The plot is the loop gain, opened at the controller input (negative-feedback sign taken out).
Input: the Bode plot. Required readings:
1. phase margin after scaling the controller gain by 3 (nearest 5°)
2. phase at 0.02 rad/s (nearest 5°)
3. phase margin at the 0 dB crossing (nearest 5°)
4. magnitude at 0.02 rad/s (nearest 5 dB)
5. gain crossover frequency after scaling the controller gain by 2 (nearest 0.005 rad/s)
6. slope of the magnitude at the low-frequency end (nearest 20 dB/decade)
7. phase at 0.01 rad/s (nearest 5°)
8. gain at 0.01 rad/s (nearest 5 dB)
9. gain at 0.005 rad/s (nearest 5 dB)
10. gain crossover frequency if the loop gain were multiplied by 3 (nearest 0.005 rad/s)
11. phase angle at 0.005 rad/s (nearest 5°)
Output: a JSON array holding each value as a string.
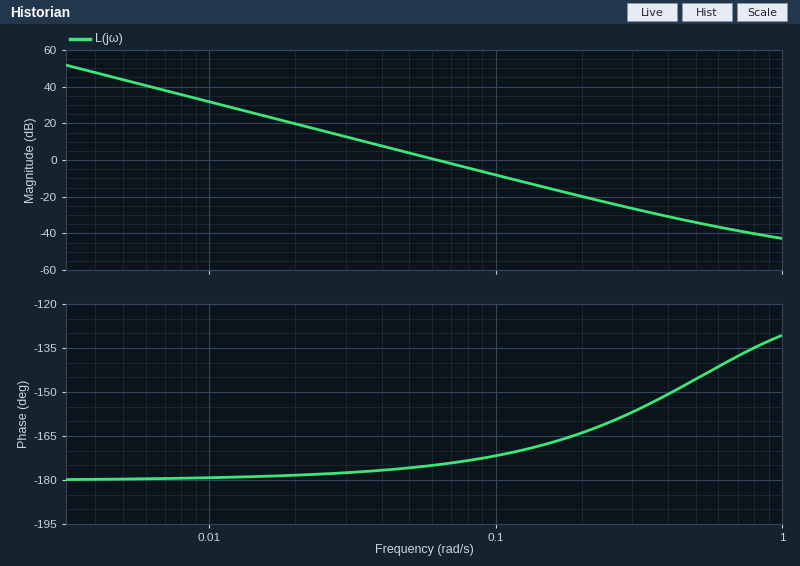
["10°", "-180°", "5°", "20 dB", "0.090 rad/s", "-40 dB/decade", "-180°", "30 dB", "45 dB", "0.110 rad/s", "-180°"]
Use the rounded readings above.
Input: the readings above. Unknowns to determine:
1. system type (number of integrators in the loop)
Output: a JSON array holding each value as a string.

["2"]
